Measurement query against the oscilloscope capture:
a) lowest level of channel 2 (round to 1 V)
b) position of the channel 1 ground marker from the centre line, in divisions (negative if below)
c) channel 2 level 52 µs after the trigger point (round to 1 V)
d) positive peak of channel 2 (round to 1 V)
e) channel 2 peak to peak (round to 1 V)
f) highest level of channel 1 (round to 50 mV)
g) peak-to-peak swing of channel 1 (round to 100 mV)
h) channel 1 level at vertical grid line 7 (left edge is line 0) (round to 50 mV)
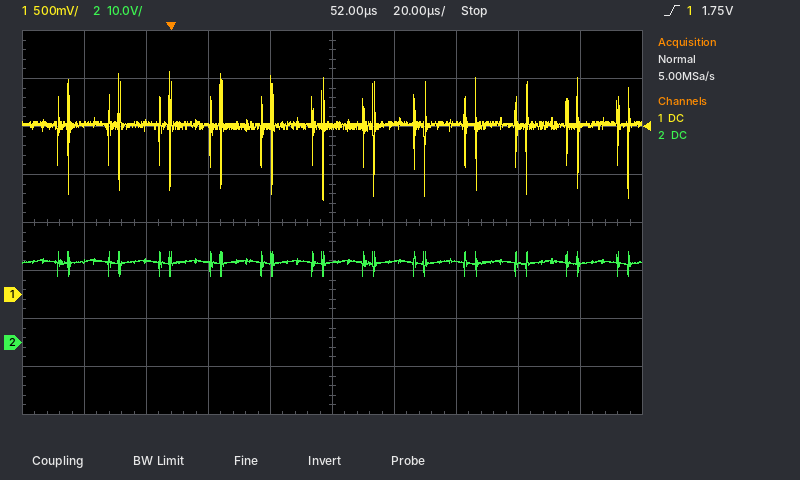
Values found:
14 V
-1.5 div
17 V
19 V
5 V
2.30 V
1.30 V
1.80 V
